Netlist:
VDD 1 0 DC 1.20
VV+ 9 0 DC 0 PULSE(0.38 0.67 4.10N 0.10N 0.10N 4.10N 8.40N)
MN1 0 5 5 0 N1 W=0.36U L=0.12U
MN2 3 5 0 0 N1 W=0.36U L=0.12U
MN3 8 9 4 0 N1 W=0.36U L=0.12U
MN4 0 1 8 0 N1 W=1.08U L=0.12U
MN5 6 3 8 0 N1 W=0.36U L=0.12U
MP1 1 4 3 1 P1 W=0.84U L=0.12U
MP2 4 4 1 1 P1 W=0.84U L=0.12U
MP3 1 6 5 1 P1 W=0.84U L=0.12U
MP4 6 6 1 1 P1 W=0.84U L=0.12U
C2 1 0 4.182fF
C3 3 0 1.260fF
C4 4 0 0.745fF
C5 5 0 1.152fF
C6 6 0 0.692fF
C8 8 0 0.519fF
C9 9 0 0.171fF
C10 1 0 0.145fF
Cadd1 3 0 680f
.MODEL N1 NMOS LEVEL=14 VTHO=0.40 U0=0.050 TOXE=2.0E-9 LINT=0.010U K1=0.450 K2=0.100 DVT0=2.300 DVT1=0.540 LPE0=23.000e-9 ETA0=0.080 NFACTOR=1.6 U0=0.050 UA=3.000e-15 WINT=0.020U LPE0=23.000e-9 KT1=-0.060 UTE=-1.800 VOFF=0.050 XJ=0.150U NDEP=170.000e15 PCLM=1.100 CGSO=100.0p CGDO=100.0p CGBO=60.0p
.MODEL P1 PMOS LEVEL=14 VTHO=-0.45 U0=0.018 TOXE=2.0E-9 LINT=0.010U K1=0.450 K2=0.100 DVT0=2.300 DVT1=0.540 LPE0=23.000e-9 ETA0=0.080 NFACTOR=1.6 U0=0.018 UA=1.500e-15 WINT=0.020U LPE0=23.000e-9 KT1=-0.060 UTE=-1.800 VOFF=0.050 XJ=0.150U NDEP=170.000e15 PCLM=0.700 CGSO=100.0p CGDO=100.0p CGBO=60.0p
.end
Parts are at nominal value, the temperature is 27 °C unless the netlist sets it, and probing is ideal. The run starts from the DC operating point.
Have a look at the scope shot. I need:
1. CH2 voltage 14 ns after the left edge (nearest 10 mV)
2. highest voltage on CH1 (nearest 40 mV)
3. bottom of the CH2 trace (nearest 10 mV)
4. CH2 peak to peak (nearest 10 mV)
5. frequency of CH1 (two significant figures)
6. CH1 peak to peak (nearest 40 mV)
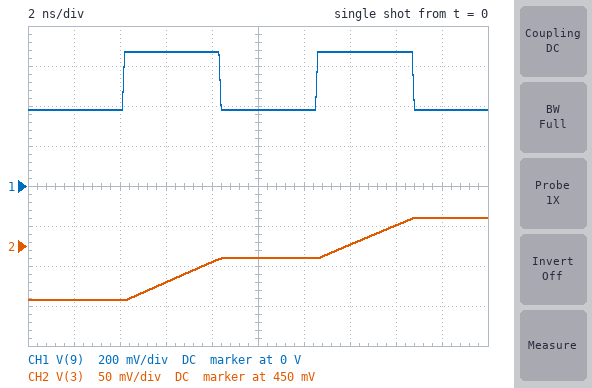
450 mV
680 mV
380 mV
100 mV
120 MHz
280 mV
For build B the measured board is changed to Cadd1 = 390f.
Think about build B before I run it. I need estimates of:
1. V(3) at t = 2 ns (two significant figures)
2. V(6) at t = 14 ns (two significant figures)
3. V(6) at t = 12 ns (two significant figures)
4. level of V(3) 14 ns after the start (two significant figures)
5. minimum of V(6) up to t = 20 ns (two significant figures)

380 mV
660 mV
680 mV
500 mV
600 mV
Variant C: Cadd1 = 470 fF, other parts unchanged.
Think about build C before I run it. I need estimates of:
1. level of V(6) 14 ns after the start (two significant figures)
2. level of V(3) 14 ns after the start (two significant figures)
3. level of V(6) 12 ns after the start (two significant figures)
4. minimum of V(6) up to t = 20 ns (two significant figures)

680 mV
480 mV
700 mV
620 mV
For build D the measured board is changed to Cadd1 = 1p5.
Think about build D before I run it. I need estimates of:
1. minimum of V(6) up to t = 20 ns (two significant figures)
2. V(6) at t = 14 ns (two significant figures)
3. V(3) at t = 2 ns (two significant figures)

720 mV
740 mV
380 mV
